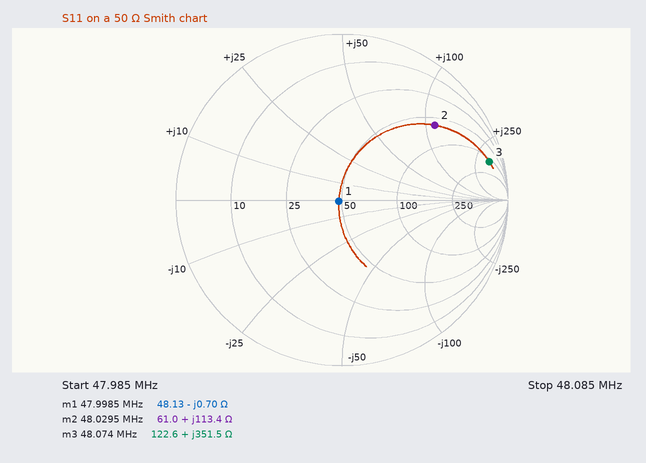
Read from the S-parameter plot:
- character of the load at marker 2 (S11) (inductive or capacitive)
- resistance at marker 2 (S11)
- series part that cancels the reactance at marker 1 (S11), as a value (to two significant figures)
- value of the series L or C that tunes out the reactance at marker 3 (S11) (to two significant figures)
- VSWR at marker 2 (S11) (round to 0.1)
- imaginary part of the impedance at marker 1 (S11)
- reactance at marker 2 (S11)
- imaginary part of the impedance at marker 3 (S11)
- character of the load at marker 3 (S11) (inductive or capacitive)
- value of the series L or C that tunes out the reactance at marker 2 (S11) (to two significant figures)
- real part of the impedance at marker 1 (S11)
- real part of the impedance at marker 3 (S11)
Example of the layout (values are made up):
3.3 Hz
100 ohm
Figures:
inductive
61.0 Ω
2.3 nH
9.4 pF
6.1
-0.70 Ω
+113.4 Ω
+351.5 Ω
inductive
29 pF
48.13 Ω
122.6 Ω
